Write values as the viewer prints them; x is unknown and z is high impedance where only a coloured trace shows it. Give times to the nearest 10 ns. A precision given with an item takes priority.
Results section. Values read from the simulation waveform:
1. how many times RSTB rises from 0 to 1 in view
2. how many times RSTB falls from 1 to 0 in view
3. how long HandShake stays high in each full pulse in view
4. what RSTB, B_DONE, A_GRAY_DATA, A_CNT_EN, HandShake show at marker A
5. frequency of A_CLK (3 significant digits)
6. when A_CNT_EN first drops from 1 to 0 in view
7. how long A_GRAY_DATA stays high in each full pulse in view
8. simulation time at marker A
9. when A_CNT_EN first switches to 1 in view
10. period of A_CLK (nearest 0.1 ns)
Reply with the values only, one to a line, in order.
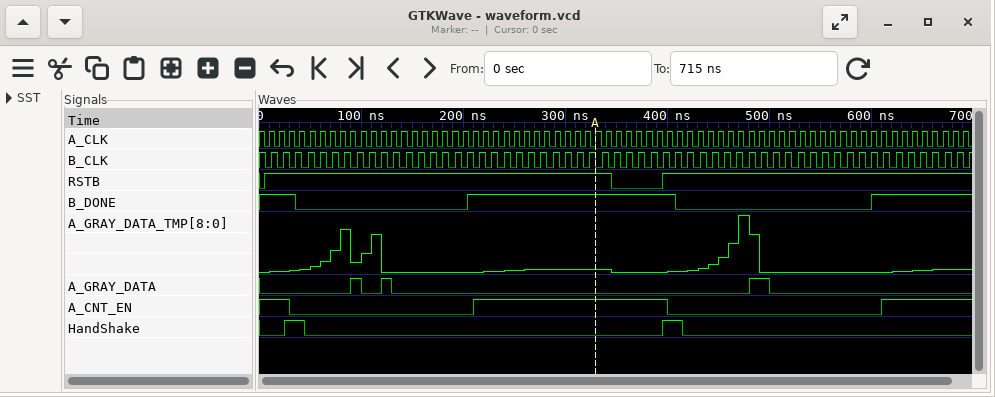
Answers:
2
1
20 ns, 20 ns
RSTB=1, B_DONE=1, A_GRAY_DATA=0, A_CNT_EN=1, HandShake=0
100 MHz
30 ns
10 ns, 10 ns, 20 ns
330 ns
210 ns
10 ns
